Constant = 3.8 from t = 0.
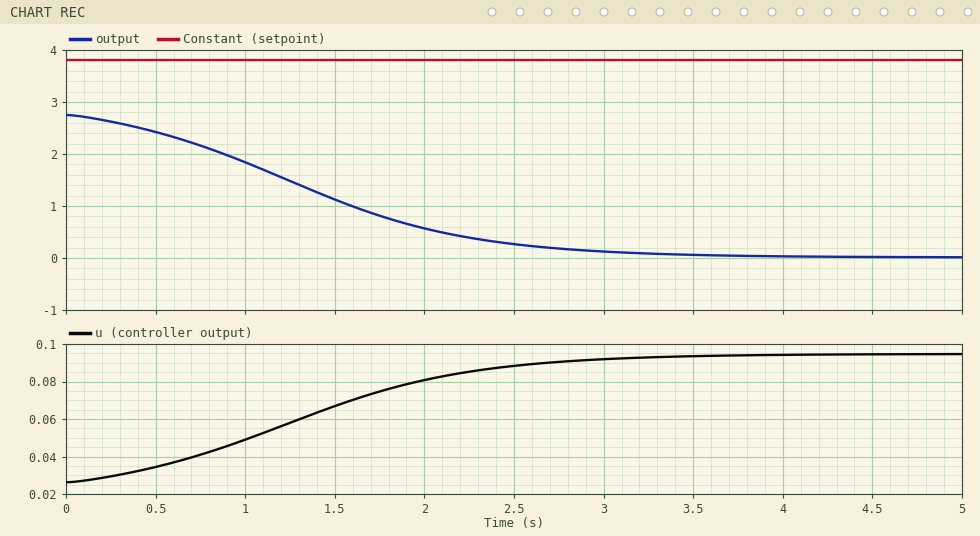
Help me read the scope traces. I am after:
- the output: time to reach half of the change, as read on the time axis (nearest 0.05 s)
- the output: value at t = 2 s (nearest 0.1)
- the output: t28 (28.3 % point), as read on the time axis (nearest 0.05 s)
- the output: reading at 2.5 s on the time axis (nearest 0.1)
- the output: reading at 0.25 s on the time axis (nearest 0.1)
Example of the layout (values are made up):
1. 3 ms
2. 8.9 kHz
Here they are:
1. 1.30 s
2. 0.6
3. 0.90 s
4. 0.3
5. 2.6
